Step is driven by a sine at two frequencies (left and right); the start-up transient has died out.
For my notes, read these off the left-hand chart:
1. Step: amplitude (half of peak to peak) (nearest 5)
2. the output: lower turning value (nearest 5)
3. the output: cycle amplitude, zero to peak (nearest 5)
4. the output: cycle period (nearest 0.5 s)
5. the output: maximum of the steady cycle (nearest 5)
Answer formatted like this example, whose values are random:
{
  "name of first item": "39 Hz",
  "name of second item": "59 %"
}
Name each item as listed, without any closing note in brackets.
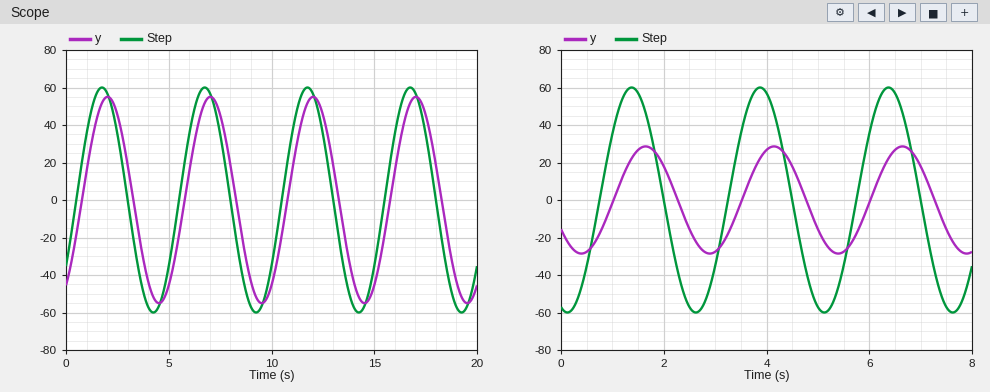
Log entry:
{
  "Step: amplitude (half of peak to peak)": "60",
  "the output: lower turning value": "-55",
  "the output: cycle amplitude, zero to peak": "55",
  "the output: cycle period": "5.0 s",
  "the output: maximum of the steady cycle": "55"
}
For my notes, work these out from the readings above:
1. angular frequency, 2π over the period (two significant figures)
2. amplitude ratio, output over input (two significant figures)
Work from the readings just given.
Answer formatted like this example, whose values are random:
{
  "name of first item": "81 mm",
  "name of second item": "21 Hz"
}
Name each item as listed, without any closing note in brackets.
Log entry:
{
  "angular frequency, 2π over the period": "1.3 rad/s",
  "amplitude ratio, output over input": "0.92"
}
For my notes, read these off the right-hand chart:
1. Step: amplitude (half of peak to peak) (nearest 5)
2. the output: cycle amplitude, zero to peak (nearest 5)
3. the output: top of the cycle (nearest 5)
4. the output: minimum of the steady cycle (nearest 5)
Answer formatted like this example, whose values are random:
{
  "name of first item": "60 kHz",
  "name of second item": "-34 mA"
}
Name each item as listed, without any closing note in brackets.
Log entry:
{
  "Step: amplitude (half of peak to peak)": "60",
  "the output: cycle amplitude, zero to peak": "30",
  "the output: top of the cycle": "30",
  "the output: minimum of the steady cycle": "-30"
}
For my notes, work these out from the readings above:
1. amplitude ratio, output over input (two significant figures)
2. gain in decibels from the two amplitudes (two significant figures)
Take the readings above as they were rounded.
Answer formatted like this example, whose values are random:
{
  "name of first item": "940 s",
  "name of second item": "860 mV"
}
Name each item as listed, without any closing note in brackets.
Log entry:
{
  "amplitude ratio, output over input": "0.50",
  "gain in decibels from the two amplitudes": "-6.0 dB"
}
